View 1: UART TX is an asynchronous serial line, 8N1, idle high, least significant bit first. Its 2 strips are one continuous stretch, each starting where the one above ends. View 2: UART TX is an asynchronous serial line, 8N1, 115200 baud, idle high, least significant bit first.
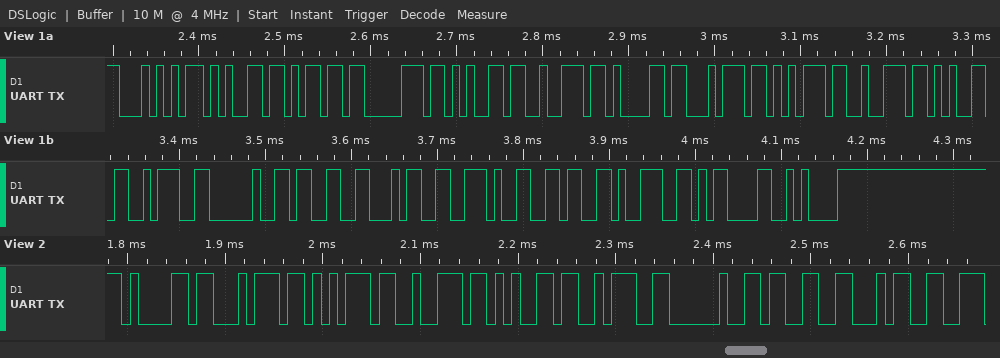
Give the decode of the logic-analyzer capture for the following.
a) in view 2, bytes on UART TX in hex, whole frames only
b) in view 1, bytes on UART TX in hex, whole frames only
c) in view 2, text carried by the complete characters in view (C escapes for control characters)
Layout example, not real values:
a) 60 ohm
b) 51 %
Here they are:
a) 0x61 0x74 0x75 0x72 0x65 0x3A 0x20 0x33 0x34
b) 54 65 6D 70 65 72 61 74 75 72 65 3A 20 33 34 2E 36 39 0D 0A
c) "ature: 34"
